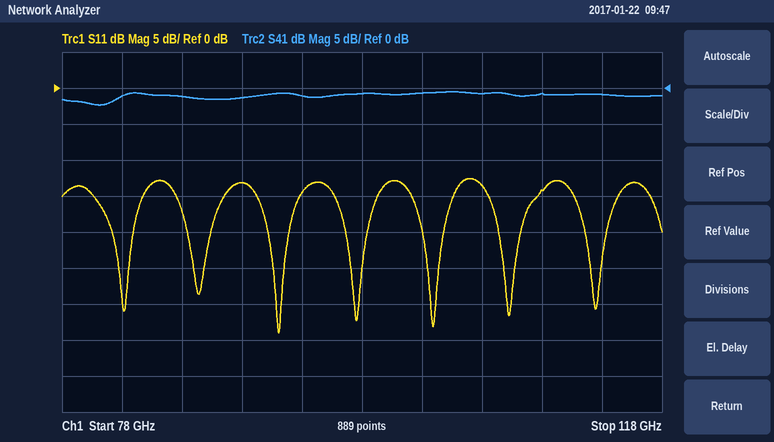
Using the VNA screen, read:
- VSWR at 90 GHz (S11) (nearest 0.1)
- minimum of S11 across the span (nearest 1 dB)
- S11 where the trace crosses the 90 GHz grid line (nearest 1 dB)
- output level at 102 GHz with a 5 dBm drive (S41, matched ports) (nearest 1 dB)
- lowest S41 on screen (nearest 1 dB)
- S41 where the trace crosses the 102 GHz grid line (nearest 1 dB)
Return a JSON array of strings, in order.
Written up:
["1.6", "-34 dB", "-13 dB", "4 dBm", "-2 dB", "-1 dB"]
